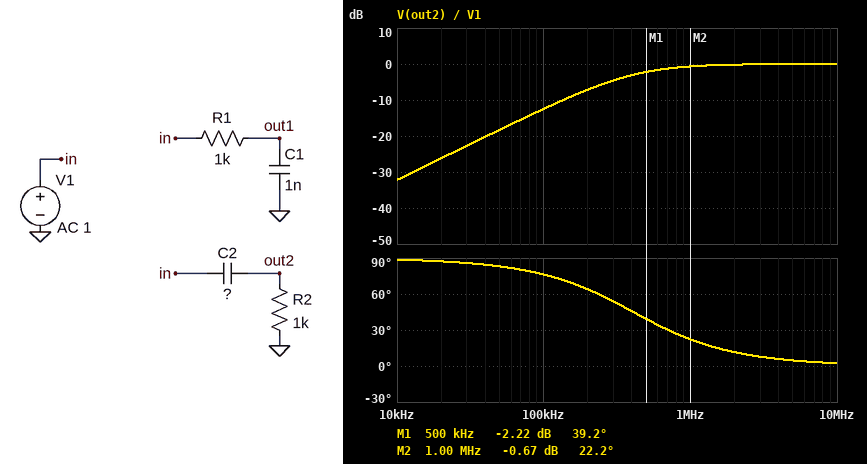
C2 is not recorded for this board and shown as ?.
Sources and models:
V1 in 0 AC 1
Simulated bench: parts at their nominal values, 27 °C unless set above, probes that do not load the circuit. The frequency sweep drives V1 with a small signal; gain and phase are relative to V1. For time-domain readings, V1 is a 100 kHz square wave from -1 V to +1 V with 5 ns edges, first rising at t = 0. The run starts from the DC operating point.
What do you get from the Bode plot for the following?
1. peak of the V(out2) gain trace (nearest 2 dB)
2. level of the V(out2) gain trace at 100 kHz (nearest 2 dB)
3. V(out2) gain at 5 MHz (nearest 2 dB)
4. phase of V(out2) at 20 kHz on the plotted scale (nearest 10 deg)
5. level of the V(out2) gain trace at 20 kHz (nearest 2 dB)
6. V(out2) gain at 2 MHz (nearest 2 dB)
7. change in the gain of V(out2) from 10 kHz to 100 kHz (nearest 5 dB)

0 dB
-12 dB
0 dB
90 deg
-26 dB
0 dB
20 dB
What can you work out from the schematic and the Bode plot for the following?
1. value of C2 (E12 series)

390 pF
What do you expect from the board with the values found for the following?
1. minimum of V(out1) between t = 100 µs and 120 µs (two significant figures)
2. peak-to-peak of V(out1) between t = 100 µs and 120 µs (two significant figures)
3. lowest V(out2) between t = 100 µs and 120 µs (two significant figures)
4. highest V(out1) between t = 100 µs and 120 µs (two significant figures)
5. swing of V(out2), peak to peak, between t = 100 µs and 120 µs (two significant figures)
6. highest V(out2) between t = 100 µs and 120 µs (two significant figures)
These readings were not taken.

-990 mV
2.0 V
-2.0 V
990 mV
4.0 V
2.0 V
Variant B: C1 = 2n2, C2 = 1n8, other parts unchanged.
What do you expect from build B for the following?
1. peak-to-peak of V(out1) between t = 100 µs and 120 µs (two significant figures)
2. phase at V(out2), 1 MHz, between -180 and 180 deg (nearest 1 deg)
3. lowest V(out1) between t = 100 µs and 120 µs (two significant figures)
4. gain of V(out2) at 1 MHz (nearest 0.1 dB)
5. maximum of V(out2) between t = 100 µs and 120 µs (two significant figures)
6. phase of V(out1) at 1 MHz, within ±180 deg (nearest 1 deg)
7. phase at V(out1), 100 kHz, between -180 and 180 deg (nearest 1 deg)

1.6 V
5 deg
-810 mV
0 dB
1.9 V
-86 deg
-54 deg
